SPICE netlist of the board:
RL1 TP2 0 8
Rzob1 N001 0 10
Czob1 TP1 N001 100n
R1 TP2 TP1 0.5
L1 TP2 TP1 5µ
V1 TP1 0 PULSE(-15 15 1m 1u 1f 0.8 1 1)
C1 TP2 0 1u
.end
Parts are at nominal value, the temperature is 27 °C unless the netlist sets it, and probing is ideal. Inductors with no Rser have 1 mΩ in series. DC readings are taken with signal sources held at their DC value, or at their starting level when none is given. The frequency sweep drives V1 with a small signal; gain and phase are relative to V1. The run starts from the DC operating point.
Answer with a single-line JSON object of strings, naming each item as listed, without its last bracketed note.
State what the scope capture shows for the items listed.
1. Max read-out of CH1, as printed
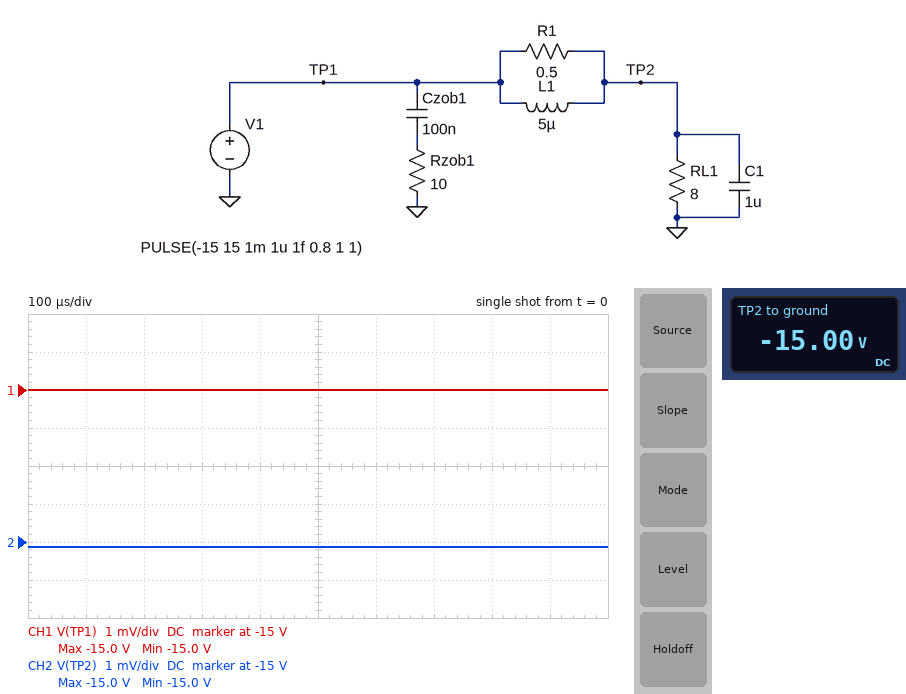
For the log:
{"Max read-out of CH1, as printed": "-15.0 V"}
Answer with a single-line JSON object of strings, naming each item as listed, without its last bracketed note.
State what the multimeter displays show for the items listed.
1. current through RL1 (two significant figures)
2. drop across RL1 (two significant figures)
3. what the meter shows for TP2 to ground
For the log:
{"current through RL1": "1.9 A", "drop across RL1": "15 V", "what the meter shows for TP2 to ground": "-15.00 V"}
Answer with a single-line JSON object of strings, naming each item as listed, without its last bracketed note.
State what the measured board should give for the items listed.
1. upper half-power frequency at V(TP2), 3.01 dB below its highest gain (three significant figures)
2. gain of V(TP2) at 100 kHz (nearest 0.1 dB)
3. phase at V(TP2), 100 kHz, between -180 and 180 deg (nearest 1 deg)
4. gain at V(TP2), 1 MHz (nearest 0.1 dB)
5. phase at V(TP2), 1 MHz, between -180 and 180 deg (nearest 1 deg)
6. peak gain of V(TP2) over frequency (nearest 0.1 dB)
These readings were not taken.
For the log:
{"upper half-power frequency at V(TP2), 3.01 dB below its highest gain": "314 kHz", "gain of V(TP2) at 100 kHz": "-0.5 dB", "phase at V(TP2), 100 kHz, between -180 and 180 deg": "-17 deg", "gain at V(TP2), 1 MHz": "-10.4 dB", "phase at V(TP2), 1 MHz, between -180 and 180 deg": "-72 deg", "peak gain of V(TP2) over frequency": "0 dB"}
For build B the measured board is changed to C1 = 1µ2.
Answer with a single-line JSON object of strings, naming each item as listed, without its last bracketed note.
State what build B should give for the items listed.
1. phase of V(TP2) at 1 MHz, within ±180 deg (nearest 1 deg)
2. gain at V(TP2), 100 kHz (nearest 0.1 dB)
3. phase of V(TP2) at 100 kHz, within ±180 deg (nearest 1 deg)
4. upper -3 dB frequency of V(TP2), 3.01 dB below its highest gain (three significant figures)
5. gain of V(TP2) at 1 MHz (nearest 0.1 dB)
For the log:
{"phase of V(TP2) at 1 MHz, within ±180 deg": "-75 deg", "gain at V(TP2), 100 kHz": "-0.6 dB", "phase of V(TP2) at 100 kHz, within ±180 deg": "-21 deg", "upper -3 dB frequency of V(TP2), 3.01 dB below its highest gain": "265 kHz", "gain of V(TP2) at 1 MHz": "-11.8 dB"}
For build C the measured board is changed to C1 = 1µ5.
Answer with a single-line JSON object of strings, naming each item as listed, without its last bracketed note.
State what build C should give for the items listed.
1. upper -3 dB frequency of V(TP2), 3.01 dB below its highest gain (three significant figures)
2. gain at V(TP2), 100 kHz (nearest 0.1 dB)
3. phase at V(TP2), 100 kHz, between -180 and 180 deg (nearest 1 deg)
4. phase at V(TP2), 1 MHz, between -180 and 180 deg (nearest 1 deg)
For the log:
{"upper -3 dB frequency of V(TP2), 3.01 dB below its highest gain": "213 kHz", "gain at V(TP2), 100 kHz": "-0.8 dB", "phase at V(TP2), 100 kHz, between -180 and 180 deg": "-25 deg", "phase at V(TP2), 1 MHz, between -180 and 180 deg": "-78 deg"}
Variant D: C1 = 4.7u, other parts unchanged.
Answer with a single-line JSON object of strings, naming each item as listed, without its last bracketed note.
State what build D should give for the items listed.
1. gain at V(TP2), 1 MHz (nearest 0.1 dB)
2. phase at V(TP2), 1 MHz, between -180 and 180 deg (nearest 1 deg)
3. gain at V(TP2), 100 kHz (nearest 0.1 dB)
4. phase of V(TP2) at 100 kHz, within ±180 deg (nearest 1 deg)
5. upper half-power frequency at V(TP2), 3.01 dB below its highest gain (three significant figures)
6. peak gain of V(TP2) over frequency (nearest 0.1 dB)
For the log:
{"gain at V(TP2), 1 MHz": "-23.4 dB", "phase at V(TP2), 1 MHz, between -180 and 180 deg": "-87 deg", "gain at V(TP2), 100 kHz": "-4.5 dB", "phase of V(TP2) at 100 kHz, within ±180 deg": "-60 deg", "upper half-power frequency at V(TP2), 3.01 dB below its highest gain": "69.9 kHz", "peak gain of V(TP2) over frequency": "0.7 dB"}
